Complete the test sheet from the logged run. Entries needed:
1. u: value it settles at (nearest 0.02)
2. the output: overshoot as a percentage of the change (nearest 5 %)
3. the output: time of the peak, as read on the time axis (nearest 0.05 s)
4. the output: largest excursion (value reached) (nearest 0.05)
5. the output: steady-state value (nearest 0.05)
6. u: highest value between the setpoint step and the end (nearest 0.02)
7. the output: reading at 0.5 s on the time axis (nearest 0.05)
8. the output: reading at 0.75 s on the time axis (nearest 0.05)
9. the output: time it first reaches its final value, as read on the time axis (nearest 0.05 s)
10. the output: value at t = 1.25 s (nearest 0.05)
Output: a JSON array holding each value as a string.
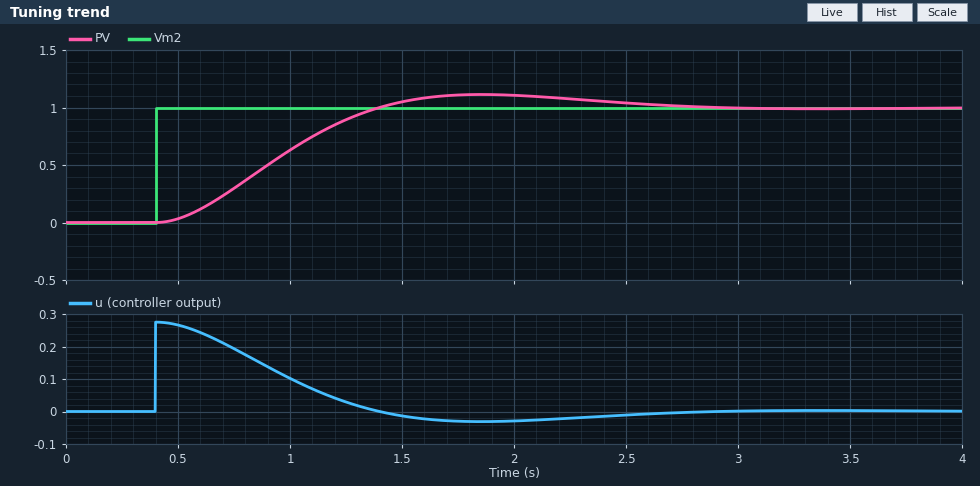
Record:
["0.00", "10 %", "1.85 s", "1.10", "1.00", "0.28", "0.05", "0.30", "1.40 s", "0.90"]
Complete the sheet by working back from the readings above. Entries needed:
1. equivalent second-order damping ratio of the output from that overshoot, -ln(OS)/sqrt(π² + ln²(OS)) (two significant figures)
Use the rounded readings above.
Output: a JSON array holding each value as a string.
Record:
["0.59"]
